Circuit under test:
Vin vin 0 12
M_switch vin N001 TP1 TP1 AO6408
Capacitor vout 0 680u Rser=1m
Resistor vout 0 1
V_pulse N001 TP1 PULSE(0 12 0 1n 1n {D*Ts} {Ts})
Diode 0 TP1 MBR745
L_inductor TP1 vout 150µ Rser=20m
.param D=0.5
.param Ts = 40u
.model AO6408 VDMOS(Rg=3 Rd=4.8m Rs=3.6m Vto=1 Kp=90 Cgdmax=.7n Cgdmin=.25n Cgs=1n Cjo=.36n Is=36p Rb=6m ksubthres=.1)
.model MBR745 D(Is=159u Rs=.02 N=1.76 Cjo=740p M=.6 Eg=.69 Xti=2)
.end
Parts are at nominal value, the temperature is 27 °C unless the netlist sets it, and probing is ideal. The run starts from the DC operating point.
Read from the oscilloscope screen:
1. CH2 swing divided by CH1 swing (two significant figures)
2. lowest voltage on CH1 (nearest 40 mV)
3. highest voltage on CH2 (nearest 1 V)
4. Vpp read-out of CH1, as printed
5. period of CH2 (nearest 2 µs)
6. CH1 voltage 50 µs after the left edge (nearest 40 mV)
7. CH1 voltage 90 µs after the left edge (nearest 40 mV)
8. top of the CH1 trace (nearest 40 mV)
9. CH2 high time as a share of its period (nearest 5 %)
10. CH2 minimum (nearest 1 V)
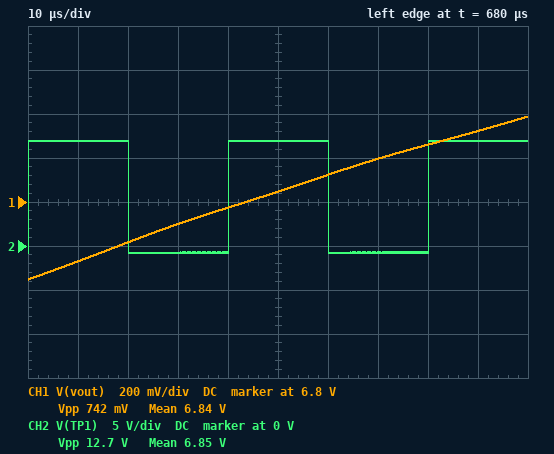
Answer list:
17
6.44 V
12 V
742 mV
40 µs
6.84 V
7.12 V
7.20 V
50 %
-1 V
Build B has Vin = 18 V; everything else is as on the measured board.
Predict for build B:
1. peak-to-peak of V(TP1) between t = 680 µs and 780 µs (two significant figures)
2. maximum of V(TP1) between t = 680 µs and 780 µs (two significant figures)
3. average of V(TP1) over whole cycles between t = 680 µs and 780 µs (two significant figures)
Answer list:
19 V
18 V
8.5 V
